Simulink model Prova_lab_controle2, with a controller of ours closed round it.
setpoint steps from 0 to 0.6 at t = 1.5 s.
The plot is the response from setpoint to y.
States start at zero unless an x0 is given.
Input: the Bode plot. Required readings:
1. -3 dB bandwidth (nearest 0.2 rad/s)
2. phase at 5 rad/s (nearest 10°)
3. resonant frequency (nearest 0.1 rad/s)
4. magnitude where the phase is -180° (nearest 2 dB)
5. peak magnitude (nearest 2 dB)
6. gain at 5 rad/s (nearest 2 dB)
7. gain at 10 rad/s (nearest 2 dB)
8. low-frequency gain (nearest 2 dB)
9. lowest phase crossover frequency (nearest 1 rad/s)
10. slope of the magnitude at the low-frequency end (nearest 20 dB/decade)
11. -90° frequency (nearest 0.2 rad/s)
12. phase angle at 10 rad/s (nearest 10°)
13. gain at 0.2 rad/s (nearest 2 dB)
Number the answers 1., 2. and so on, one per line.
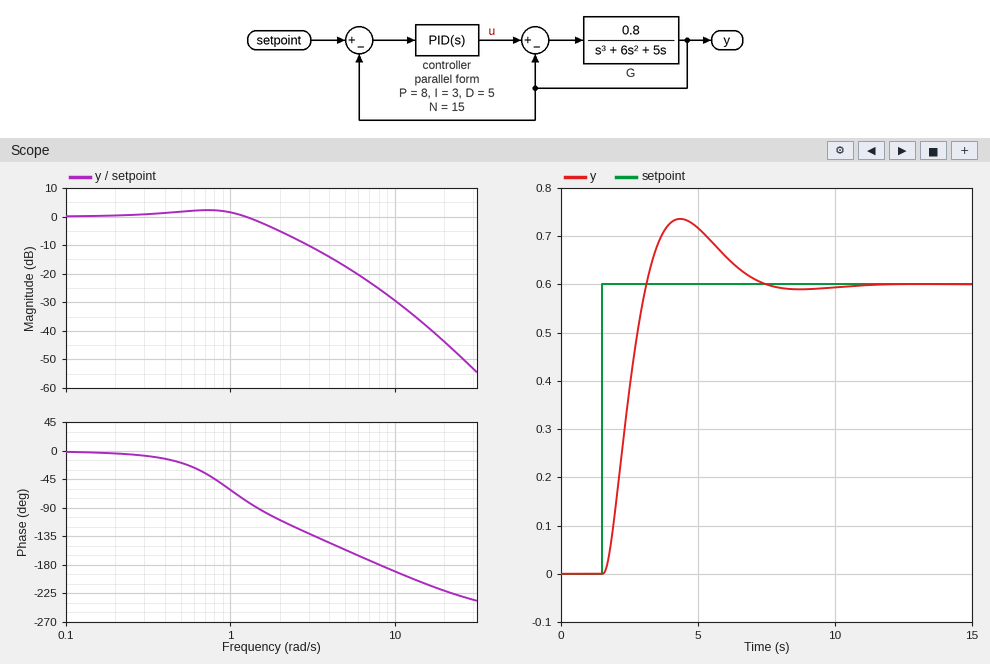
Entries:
1. 1.6 rad/s
2. -160°
3. 0.7 rad/s
4. -26 dB
5. 2 dB
6. -18 dB
7. -30 dB
8. 0 dB
9. 8 rad/s
10. 0 dB/decade
11. 1.4 rad/s
12. -190°
13. 0 dB
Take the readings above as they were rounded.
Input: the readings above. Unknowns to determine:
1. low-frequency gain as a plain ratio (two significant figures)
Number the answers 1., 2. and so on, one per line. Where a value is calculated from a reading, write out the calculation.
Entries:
1. 10^(0 / 20) = 1.0
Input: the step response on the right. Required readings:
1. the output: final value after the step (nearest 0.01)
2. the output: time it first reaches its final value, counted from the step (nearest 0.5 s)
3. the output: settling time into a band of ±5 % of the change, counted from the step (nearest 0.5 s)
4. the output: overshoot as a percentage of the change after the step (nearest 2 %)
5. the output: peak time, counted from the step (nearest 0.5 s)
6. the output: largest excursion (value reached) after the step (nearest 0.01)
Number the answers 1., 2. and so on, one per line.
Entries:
1. 0.60
2. 1.5 s
3. 5.0 s
4. 22 %
5. 3.0 s
6. 0.74
